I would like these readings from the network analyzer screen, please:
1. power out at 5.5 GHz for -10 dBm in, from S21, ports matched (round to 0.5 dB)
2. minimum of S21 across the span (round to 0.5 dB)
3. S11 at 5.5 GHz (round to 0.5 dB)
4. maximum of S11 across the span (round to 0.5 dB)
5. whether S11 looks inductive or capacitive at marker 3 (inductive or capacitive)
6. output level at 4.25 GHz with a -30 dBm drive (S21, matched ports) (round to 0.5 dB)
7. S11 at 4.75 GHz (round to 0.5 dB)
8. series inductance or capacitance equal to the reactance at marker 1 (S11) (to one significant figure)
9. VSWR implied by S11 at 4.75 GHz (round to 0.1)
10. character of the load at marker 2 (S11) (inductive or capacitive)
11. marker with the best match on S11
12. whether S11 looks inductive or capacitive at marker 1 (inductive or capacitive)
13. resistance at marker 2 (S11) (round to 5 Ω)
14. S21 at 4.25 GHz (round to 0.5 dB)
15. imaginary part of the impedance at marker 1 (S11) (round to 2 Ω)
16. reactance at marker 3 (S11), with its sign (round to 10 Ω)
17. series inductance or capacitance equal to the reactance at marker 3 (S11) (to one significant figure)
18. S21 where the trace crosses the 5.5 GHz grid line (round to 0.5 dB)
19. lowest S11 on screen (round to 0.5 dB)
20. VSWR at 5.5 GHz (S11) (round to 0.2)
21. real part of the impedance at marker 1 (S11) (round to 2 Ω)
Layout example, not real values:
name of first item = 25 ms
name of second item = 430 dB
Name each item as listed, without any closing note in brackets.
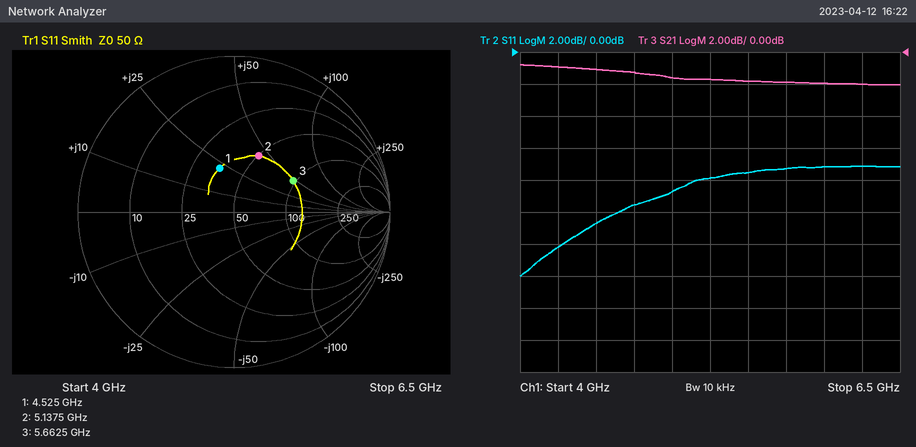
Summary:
power out at 5.5 GHz for -10 dBm in, from S21, ports matched = -12.0 dBm
minimum of S21 across the span = -2.0 dB
S11 at 5.5 GHz = -7.5 dB
maximum of S11 across the span = -7.0 dB
whether S11 looks inductive or capacitive at marker 3 = inductive
output level at 4.25 GHz with a -30 dBm drive (S21, matched ports) = -31.0 dBm
S11 at 4.75 GHz = -9.5 dB
series inductance or capacitance equal to the reactance at marker 1 (S11) = 800 pH
VSWR implied by S11 at 4.75 GHz = 2.0
character of the load at marker 2 (S11) = inductive
marker with the best match on S11 = marker 1
whether S11 looks inductive or capacitive at marker 1 = inductive
resistance at marker 2 (S11) = 50 Ω
S21 at 4.25 GHz = -1.0 dB
imaginary part of the impedance at marker 1 (S11) = +22 Ω
reactance at marker 3 (S11), with its sign = +50 Ω
series inductance or capacitance equal to the reactance at marker 3 (S11) = 1 nH
S21 where the trace crosses the 5.5 GHz grid line = -2.0 dB
lowest S11 on screen = -14.0 dB
VSWR at 5.5 GHz (S11) = 2.4
real part of the impedance at marker 1 (S11) = 36 Ω
